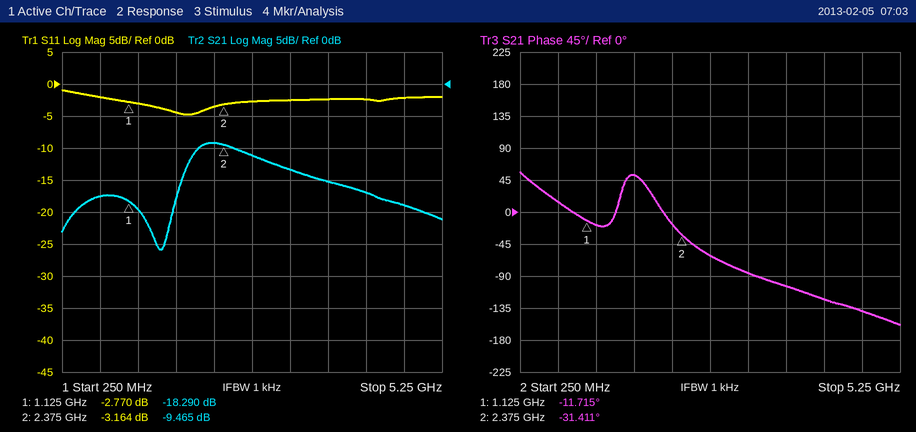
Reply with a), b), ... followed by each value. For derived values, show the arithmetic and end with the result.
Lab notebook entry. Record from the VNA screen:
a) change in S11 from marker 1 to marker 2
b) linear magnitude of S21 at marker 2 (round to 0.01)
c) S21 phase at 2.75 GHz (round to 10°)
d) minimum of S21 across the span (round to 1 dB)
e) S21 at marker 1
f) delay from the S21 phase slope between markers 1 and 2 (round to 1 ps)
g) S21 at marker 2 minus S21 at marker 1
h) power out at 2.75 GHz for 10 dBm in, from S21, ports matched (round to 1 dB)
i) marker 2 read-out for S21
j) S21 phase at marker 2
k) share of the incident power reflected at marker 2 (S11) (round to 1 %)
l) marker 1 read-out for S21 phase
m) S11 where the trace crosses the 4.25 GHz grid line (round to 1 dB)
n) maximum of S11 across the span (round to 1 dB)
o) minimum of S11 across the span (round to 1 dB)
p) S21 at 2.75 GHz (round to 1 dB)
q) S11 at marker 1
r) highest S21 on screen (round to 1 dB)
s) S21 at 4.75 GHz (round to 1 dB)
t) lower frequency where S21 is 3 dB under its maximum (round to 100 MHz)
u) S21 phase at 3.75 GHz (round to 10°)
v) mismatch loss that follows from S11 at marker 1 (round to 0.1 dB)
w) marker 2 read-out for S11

a) -3.164 − (-2.77) = -0.394 dB
b) 10^(-9.465/20) ≈ 0.34
c) -60°
d) -26 dB
e) -18.290 dB
f) −(-31.411° − (-11.715°))/(360° × 1.25 GHz) ≈ 44 ps
g) -9.465 − (-18.29) = 8.825 dB
h) 10 dBm + (-11 dB) = -1 dBm
i) -9.465 dB
j) -31.411°
k) 10^(-3.164/10) ≈ 48 %
l) -11.715°
m) -2 dB
n) -1 dB
o) -5 dB
p) -11 dB
q) -2.770 dB
r) -9 dB
s) -19 dB
t) 1.9 GHz
u) -100°
v) −10 log10(1 − 10^(-2.77/10)) ≈ 3.3 dB
w) -3.164 dB
